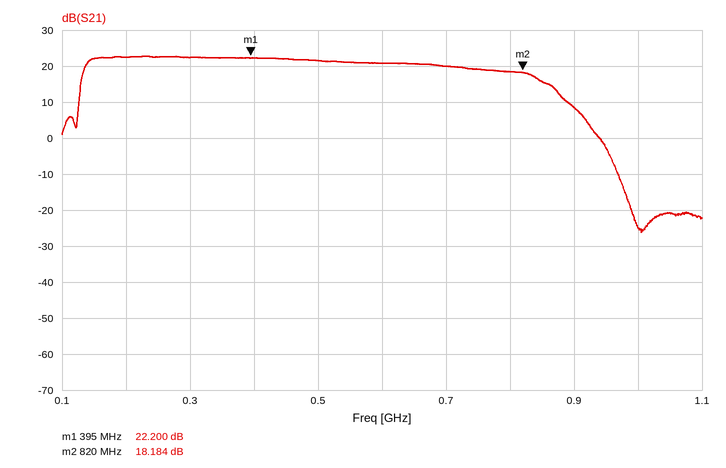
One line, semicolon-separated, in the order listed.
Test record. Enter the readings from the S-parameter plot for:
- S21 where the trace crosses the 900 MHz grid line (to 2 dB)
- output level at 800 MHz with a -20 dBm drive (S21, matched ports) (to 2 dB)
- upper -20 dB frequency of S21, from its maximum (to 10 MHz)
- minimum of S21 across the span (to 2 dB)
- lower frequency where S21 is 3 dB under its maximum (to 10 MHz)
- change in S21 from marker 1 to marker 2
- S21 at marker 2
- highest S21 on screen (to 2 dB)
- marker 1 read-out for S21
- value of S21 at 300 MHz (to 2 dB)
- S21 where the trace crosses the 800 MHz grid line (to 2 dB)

8 dB; -2 dBm; 930 MHz; -26 dB; 140 MHz; -4.016 dB; 18.184 dB; 22 dB; 22.200 dB; 22 dB; 18 dB
